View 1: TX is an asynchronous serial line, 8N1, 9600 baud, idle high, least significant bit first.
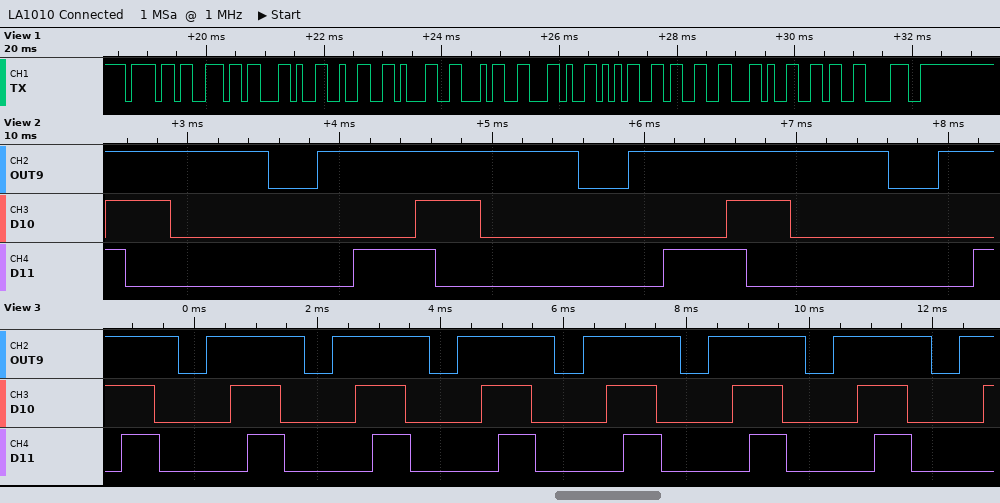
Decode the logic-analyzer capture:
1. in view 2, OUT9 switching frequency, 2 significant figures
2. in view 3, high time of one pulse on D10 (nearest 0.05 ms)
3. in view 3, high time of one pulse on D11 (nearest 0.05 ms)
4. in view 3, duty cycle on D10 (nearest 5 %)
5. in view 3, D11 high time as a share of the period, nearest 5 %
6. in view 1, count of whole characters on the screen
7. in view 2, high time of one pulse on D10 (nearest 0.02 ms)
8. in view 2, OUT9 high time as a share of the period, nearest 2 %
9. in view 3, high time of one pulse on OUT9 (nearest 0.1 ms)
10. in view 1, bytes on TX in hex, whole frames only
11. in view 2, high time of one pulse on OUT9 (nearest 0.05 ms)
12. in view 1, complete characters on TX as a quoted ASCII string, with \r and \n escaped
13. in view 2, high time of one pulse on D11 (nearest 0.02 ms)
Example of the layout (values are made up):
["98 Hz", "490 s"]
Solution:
["490 Hz", "0.80 ms", "0.60 ms", "40 %", "30 %", "12", "0.42 ms", "84 %", "1.6 ms", "6F 6E 2C 32 31 34 2C 35 33 2C 36 38", "1.70 ms", "\"on,214,53,68\"", "0.54 ms"]
